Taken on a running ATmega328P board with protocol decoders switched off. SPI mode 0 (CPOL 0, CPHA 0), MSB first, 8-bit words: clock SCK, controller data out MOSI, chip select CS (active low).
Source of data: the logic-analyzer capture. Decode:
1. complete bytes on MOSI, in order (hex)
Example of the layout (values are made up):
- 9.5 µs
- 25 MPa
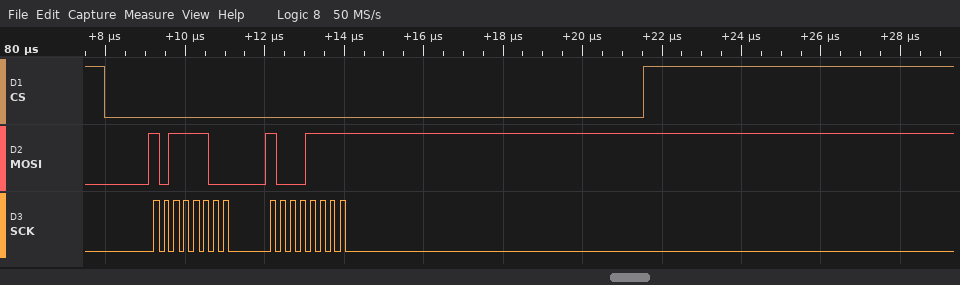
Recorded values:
- 0xBC 0x8F
